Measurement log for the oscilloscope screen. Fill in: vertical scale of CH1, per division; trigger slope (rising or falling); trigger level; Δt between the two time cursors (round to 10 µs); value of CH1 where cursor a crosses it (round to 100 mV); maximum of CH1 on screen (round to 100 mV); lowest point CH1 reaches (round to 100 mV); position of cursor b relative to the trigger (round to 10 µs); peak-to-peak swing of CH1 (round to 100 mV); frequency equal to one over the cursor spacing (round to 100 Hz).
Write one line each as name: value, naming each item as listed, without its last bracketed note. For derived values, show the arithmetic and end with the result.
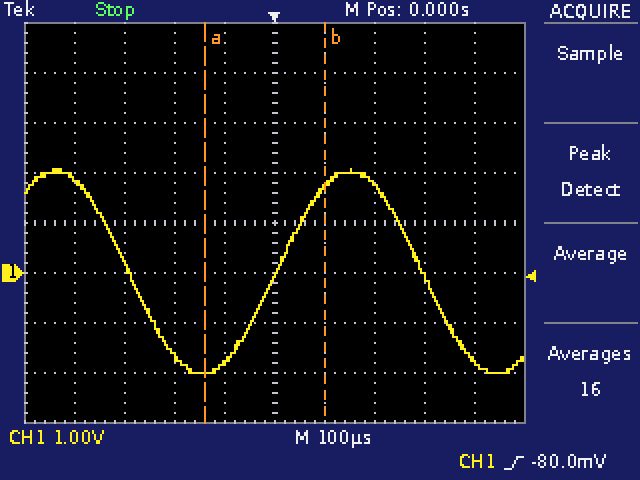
vertical scale of CH1, per division: 1 V
trigger slope: rising
trigger level: -80.0 mV
Δt between the two time cursors: 240 µs
value of CH1 where cursor a crosses it: -2.0 V
maximum of CH1 on screen: 2.1 V
lowest point CH1 reaches: -2.0 V
position of cursor b relative to the trigger: +100 µs
peak-to-peak swing of CH1: 2.1 V − (-2.0 V) = 4.1 V
frequency equal to one over the cursor spacing: 1 / 240 µs ≈ 4.2 kHz
